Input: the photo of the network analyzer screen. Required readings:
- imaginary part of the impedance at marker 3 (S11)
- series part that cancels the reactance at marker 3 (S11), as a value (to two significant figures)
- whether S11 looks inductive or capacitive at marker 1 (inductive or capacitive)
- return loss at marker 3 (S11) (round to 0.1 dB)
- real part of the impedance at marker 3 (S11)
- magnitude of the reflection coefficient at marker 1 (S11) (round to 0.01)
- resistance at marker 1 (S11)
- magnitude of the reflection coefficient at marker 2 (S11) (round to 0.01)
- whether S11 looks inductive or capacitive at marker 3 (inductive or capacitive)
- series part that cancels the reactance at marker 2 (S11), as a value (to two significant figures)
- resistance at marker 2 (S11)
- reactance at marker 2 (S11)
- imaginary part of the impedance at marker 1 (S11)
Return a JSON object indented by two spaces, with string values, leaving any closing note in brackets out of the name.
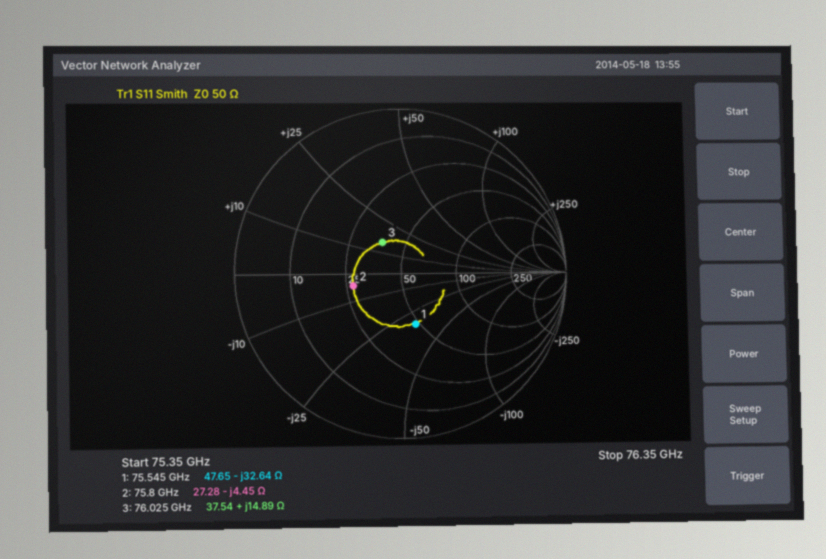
{
  "imaginary part of the impedance at marker 3": "+14.89 Ω",
  "series part that cancels the reactance at marker 3 (S11), as a value": "140 fF",
  "whether S11 looks inductive or capacitive at marker 1": "capacitive",
  "return loss at marker 3 (S11)": "13.2 dB",
  "real part of the impedance at marker 3": "37.54 Ω",
  "magnitude of the reflection coefficient at marker 1 (S11)": "0.32",
  "resistance at marker 1": "47.65 Ω",
  "magnitude of the reflection coefficient at marker 2 (S11)": "0.30",
  "whether S11 looks inductive or capacitive at marker 3": "inductive",
  "series part that cancels the reactance at marker 2 (S11), as a value": "9.3 pH",
  "resistance at marker 2": "27.28 Ω",
  "reactance at marker 2": "-4.45 Ω",
  "imaginary part of the impedance at marker 1": "-32.64 Ω"
}
